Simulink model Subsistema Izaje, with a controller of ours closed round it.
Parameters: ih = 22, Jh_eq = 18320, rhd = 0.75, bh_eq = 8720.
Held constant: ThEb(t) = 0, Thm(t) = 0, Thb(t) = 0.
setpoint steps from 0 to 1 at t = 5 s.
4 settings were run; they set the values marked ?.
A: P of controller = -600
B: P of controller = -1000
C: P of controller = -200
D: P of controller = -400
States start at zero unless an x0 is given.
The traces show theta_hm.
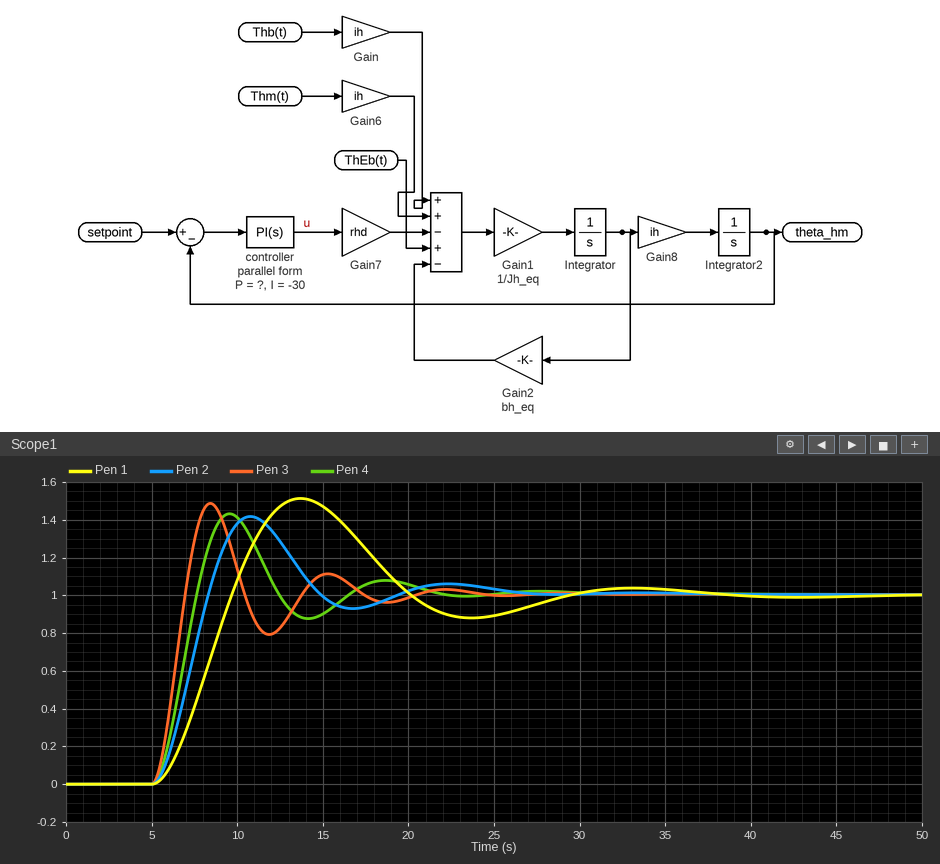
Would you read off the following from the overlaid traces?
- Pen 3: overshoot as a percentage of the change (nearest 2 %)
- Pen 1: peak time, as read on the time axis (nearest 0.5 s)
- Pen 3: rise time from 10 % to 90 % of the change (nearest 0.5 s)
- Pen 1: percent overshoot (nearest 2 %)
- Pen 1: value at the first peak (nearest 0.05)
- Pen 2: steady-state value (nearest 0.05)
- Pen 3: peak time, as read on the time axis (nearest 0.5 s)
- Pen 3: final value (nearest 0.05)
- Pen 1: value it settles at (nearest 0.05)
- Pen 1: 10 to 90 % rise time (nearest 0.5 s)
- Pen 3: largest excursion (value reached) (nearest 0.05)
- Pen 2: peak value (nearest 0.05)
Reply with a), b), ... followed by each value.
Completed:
a) 48 %
b) 13.5 s
c) 1.5 s
d) 52 %
e) 1.50
f) 1.00
g) 8.5 s
h) 1.00
i) 1.00
j) 3.0 s
k) 1.50
l) 1.40
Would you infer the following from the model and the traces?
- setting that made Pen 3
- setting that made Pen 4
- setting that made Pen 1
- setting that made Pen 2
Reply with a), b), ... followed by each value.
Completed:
a) B
b) A
c) C
d) D
